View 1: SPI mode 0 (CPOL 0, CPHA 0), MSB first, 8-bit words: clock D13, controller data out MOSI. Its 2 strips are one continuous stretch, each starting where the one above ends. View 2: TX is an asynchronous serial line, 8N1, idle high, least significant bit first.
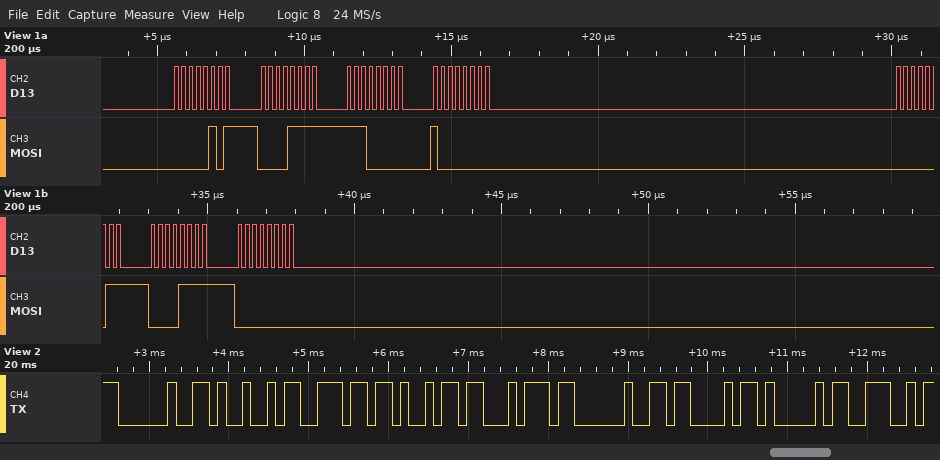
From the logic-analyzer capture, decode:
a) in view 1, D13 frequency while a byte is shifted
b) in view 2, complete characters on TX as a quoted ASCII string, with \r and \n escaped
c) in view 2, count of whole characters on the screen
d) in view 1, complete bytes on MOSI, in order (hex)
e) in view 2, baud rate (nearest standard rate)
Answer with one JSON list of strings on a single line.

["4 MHz", "\" Init CAN\"", "9", "0x05 0x0F 0xE0 0x80 0x03 0x0F 0x00", "9600 baud"]
